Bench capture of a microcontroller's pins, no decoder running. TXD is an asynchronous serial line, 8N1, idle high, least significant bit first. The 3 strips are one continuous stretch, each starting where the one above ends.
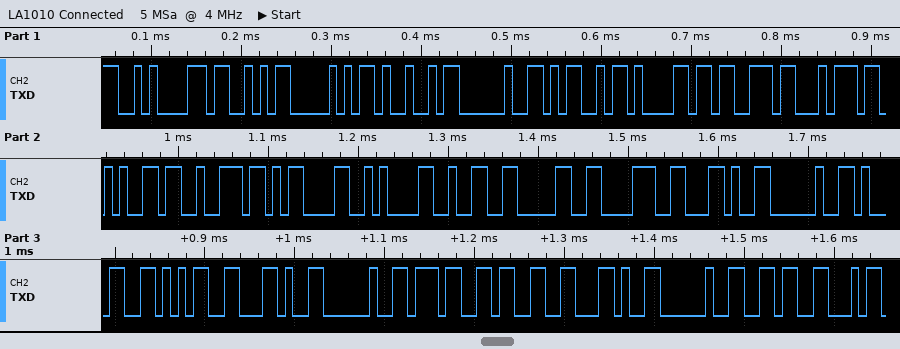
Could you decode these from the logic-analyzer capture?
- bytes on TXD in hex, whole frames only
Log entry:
0A 53 50 49 20 4D 61 73 74 65 72 0D 0A 32 30 38 2C 20 31 35 2C 20 37 33 2C 20 36
